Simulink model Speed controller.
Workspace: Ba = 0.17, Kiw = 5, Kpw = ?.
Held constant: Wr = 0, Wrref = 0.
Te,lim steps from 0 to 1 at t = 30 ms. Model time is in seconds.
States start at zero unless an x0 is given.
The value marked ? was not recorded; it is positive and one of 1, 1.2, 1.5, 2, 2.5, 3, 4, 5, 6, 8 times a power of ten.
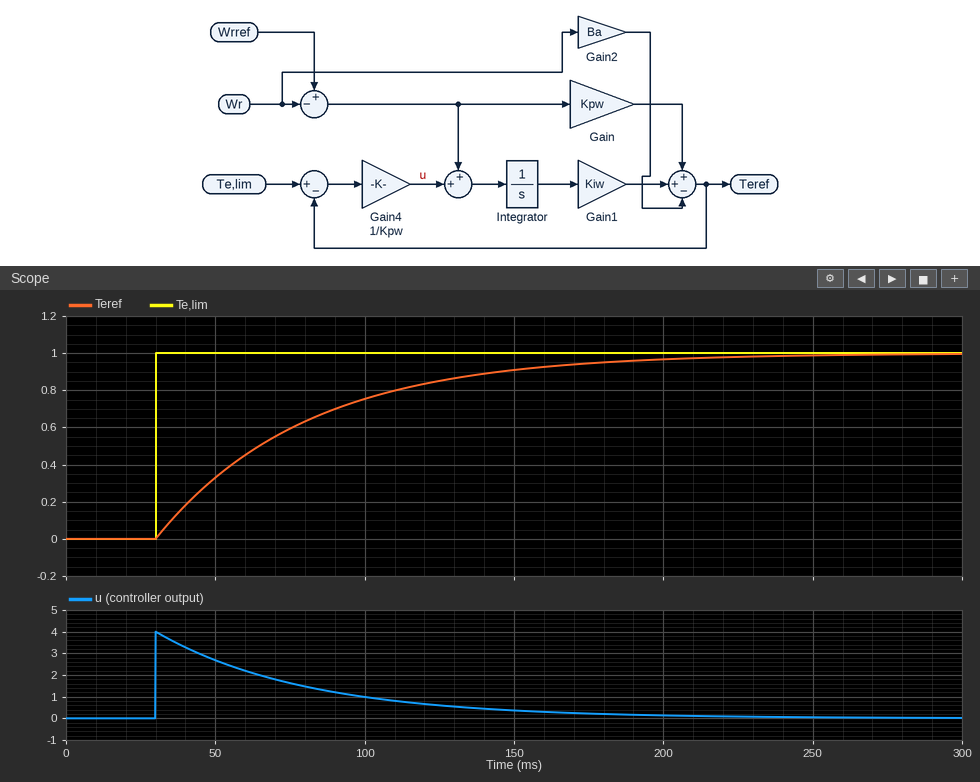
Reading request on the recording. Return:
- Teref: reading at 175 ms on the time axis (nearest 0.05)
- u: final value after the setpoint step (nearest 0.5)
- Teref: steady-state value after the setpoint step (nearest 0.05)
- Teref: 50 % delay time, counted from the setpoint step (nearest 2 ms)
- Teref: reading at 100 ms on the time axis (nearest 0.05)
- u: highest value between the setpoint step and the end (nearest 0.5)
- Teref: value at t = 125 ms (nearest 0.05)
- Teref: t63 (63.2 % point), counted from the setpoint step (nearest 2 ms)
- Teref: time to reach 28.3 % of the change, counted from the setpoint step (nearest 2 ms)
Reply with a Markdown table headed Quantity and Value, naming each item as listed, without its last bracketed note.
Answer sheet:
| Quantity | Value |
|---|---|
| Teref: reading at 175 ms on the time axis | 0.95 |
| u: final value after the setpoint step | 0.0 |
| Teref: steady-state value after the setpoint step | 1.00 |
| Teref: 50 % delay time, counted from the setpoint step | 34 ms |
| Teref: reading at 100 ms on the time axis | 0.75 |
| u: highest value between the setpoint step and the end | 4.0 |
| Teref: value at t = 125 ms | 0.85 |
| Teref: t63 (63.2 % point), counted from the setpoint step | 50 ms |
| Teref: time to reach 28.3 % of the change, counted from the setpoint step | 16 ms |
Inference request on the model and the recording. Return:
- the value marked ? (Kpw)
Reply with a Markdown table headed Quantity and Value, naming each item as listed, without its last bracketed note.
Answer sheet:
| Quantity | Value |
|---|---|
| the value marked ? | 0.25 |
